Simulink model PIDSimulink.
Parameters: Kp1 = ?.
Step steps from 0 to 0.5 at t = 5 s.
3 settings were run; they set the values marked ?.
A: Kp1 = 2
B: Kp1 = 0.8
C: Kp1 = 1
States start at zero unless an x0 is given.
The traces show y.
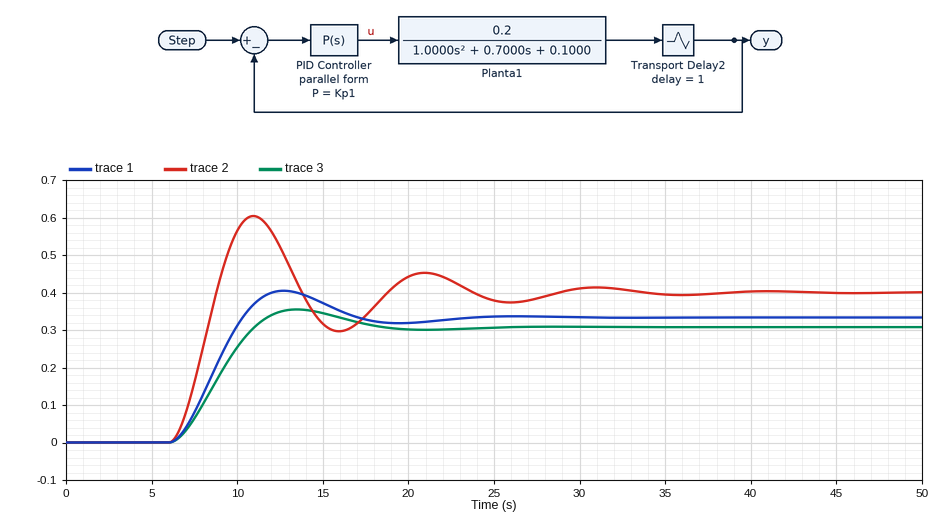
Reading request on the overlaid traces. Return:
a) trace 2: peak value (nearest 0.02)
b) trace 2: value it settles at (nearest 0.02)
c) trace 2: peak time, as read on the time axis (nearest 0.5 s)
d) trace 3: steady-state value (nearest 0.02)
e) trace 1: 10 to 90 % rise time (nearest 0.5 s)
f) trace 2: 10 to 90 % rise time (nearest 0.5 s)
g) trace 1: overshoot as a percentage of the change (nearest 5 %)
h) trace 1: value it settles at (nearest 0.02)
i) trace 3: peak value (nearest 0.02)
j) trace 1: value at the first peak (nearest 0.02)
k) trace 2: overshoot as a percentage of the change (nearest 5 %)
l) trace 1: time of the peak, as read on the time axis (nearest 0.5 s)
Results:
0.60
0.40
11.0 s
0.30
3.0 s
2.0 s
20 %
0.34
0.36
0.40
50 %
12.5 s
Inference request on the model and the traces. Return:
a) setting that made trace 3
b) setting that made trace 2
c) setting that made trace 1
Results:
B
A
C
